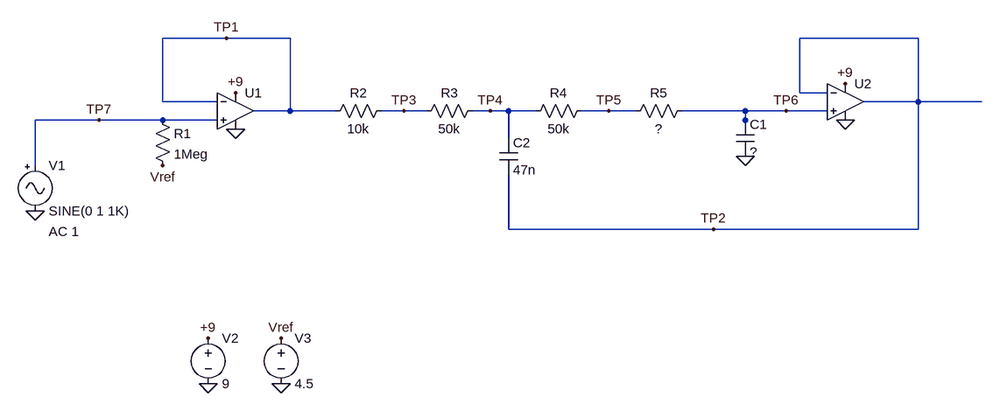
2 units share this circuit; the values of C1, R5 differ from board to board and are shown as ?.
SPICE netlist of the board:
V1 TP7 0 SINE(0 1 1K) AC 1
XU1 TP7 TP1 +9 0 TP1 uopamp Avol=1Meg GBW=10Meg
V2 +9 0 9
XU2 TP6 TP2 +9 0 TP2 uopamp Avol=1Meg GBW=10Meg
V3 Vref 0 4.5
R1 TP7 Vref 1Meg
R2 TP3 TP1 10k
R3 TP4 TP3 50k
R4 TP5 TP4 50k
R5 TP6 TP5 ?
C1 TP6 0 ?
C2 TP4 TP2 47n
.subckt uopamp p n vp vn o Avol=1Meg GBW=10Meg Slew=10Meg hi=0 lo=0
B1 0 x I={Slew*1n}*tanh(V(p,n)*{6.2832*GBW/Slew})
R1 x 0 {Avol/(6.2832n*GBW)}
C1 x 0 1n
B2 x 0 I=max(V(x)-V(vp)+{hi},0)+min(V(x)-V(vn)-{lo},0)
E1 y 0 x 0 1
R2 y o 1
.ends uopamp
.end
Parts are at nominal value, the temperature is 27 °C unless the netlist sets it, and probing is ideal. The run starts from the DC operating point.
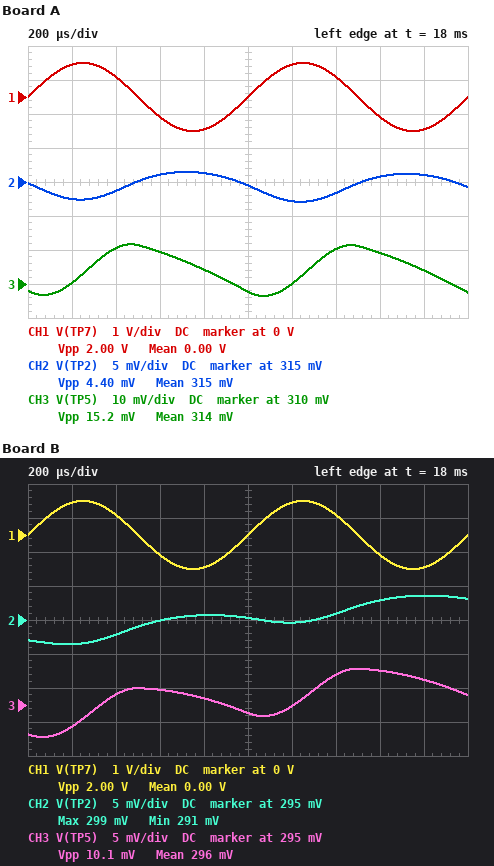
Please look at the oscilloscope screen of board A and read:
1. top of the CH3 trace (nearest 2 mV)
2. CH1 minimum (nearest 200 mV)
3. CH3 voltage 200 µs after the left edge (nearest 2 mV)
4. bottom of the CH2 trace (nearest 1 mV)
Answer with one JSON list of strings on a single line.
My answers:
["322 mV", "-1.0 V", "310 mV", "312 mV"]
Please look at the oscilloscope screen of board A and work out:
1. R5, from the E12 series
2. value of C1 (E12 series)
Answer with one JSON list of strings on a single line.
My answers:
["15 kΩ", "33 nF"]
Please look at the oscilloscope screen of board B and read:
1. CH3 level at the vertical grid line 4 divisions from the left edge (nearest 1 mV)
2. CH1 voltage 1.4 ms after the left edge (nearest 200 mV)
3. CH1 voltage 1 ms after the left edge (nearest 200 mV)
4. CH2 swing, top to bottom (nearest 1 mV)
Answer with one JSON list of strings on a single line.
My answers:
["296 mV", "600 mV", "0 V", "7 mV"]
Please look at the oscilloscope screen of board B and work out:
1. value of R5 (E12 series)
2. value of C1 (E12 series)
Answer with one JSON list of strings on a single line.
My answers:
["4.7 kΩ", "68 nF"]
